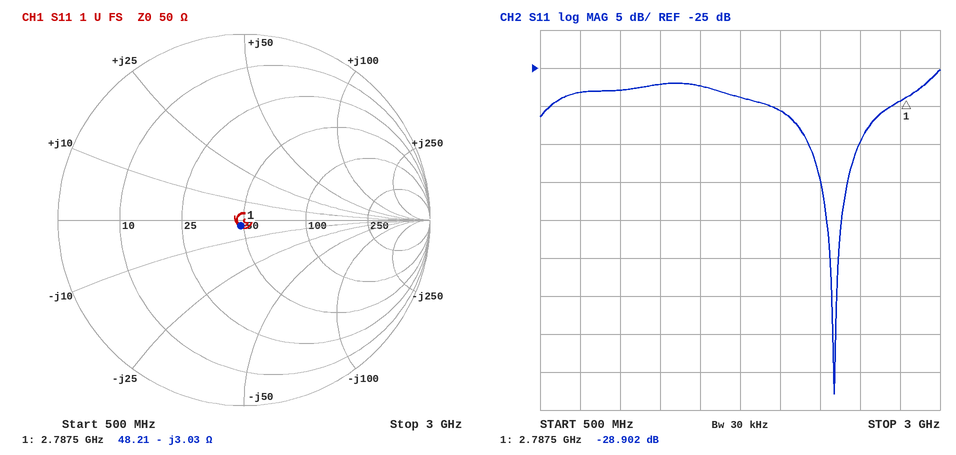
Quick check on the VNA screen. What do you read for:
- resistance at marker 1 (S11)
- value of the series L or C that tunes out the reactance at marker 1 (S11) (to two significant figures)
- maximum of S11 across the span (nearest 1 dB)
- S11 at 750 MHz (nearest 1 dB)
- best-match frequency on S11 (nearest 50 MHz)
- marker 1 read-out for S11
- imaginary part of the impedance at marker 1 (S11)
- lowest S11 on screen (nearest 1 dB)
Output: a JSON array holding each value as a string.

["48.21 Ω", "170 pH", "-25 dB", "-28 dB", "2.35 GHz", "-28.902 dB", "-3.03 Ω", "-68 dB"]
